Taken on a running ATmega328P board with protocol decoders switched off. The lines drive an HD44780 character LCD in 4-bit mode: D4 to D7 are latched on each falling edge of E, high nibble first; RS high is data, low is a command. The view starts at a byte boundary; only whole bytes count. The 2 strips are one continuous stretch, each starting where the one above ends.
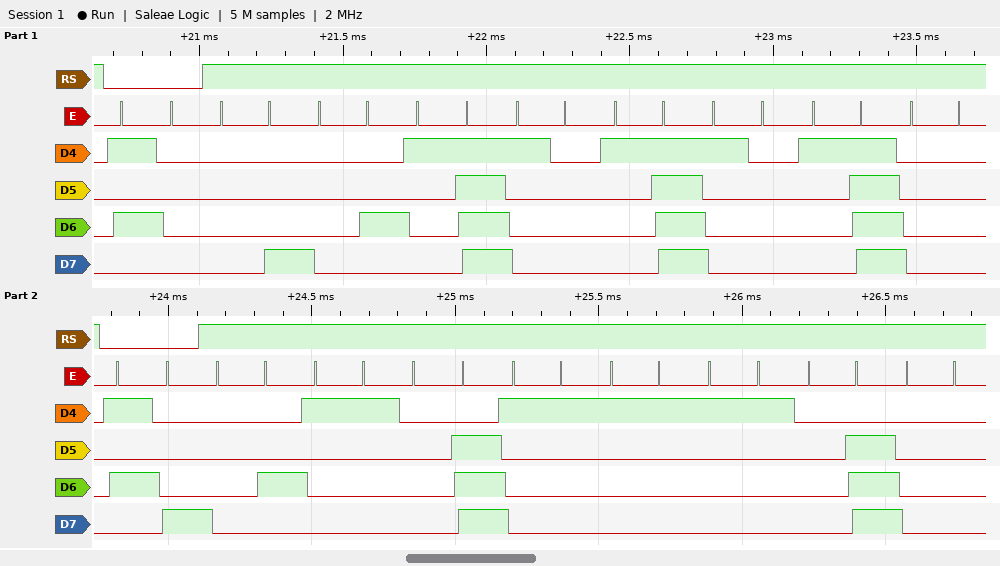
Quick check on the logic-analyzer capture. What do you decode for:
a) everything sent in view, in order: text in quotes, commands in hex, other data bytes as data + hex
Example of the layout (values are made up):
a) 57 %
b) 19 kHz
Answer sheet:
a) 0x50 data 08 04 1F 10 1F 10 1F 00 0x58 data 04 11 0E 11 11 11 0E 00
